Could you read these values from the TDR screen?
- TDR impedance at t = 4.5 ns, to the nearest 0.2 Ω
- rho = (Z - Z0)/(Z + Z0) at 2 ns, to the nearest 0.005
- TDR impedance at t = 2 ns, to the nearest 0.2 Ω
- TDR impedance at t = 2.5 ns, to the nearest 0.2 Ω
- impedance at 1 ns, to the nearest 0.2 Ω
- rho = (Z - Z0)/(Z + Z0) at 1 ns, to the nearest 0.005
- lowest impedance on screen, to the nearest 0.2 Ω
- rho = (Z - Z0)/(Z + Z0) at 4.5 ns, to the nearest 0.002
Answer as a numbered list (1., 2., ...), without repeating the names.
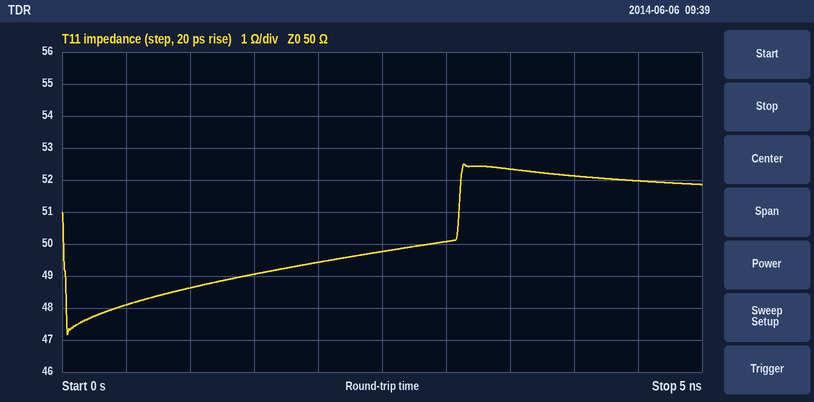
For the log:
1. 52.0 Ω
2. -0.005
3. 49.4 Ω
4. 49.8 Ω
5. 48.6 Ω
6. -0.015
7. 47.2 Ω
8. +0.020
